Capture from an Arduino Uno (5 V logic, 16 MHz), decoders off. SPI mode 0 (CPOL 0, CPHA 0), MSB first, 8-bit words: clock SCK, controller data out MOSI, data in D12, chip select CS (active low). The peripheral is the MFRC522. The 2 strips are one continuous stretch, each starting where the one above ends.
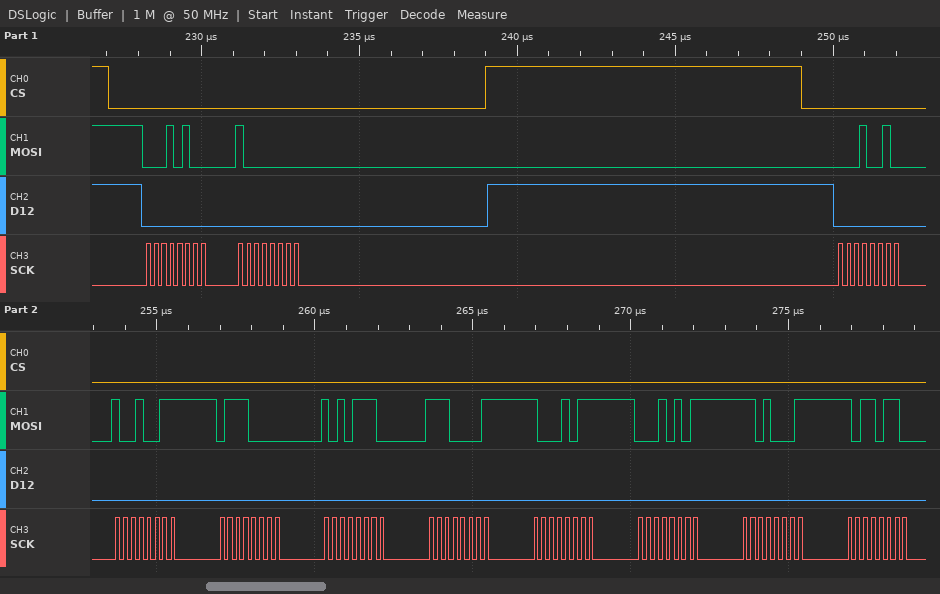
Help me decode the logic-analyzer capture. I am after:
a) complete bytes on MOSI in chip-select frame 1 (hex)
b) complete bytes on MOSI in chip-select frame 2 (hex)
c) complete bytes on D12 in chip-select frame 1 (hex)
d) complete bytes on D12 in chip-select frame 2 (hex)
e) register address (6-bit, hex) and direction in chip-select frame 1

14 80
12 93 70 AE E1 8B 15 D1 B6
00 00
00 00 00 00 00 00 00 00 00
0x0A write
